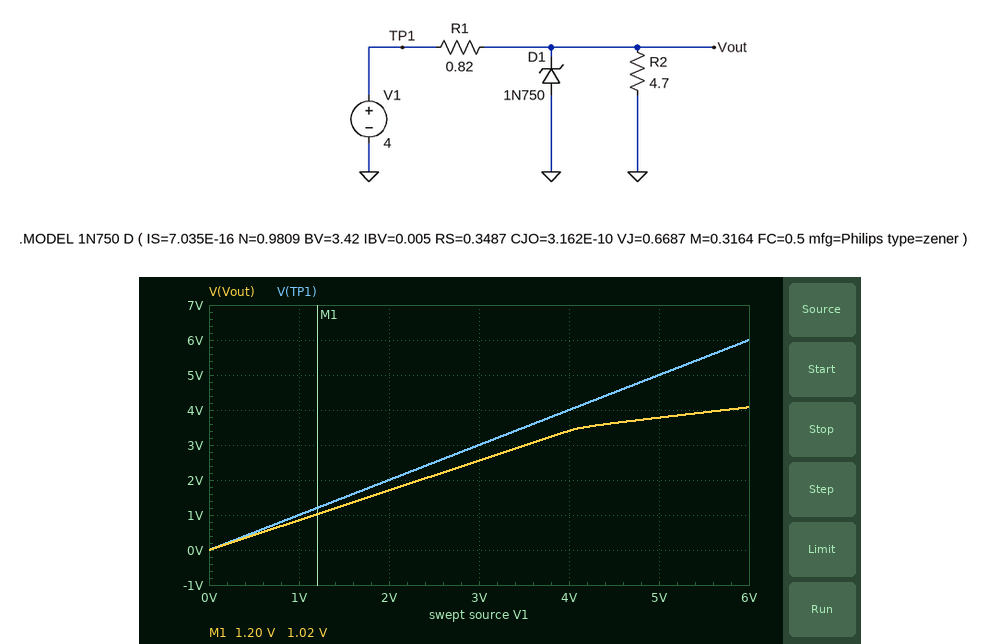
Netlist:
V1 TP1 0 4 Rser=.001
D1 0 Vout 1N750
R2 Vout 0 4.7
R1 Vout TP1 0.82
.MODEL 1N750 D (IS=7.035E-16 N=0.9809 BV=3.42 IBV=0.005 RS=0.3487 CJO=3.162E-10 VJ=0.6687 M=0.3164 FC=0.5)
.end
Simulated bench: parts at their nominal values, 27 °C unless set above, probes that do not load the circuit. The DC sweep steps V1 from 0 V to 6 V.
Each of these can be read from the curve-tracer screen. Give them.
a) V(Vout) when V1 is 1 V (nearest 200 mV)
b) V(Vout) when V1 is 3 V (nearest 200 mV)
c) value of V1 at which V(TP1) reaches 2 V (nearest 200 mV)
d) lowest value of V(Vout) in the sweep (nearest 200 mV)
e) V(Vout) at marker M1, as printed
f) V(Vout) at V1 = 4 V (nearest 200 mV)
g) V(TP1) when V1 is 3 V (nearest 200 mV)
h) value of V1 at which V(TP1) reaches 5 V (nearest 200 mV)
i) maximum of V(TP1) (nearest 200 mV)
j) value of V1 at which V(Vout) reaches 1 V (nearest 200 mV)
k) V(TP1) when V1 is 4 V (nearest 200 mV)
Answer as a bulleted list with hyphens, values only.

- 800 mV
- 2.6 V
- 2.0 V
- 0 V
- 1.02 V
- 3.4 V
- 3.0 V
- 5.0 V
- 6.0 V
- 1.2 V
- 4.0 V
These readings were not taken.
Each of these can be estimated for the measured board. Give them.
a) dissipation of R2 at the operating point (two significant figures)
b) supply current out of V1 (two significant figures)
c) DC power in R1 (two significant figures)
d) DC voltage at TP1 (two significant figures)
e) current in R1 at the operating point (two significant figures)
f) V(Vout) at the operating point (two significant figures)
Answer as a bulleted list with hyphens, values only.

- 2.5 W
- 730 mA
- 430 mW
- 4.0 V
- 730 mA
- 3.4 V
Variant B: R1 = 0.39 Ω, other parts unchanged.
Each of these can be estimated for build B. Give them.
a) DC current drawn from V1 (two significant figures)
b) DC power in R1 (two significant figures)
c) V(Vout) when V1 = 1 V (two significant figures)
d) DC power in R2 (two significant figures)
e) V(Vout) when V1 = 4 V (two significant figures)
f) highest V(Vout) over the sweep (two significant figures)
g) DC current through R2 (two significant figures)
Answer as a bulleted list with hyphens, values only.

- 1.0 A
- 400 mW
- 920 mV
- 2.8 W
- 3.6 V
- 4.5 V
- 770 mA
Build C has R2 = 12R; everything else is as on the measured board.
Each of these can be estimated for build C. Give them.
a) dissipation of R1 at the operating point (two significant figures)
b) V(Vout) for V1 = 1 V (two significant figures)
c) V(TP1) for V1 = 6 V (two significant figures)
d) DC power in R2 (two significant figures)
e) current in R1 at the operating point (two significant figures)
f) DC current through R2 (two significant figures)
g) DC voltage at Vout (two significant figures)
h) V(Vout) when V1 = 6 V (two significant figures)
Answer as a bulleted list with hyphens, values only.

- 210 mW
- 940 mV
- 6.0 V
- 1.1 W
- 500 mA
- 300 mA
- 3.6 V
- 4.2 V
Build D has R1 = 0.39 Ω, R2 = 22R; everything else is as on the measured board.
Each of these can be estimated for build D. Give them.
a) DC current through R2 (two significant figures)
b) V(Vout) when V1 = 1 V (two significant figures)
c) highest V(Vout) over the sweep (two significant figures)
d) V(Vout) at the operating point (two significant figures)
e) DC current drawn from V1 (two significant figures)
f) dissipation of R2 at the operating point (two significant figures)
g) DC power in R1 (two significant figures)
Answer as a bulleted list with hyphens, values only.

- 170 mA
- 980 mV
- 4.7 V
- 3.7 V
- 700 mA
- 630 mW
- 190 mW
